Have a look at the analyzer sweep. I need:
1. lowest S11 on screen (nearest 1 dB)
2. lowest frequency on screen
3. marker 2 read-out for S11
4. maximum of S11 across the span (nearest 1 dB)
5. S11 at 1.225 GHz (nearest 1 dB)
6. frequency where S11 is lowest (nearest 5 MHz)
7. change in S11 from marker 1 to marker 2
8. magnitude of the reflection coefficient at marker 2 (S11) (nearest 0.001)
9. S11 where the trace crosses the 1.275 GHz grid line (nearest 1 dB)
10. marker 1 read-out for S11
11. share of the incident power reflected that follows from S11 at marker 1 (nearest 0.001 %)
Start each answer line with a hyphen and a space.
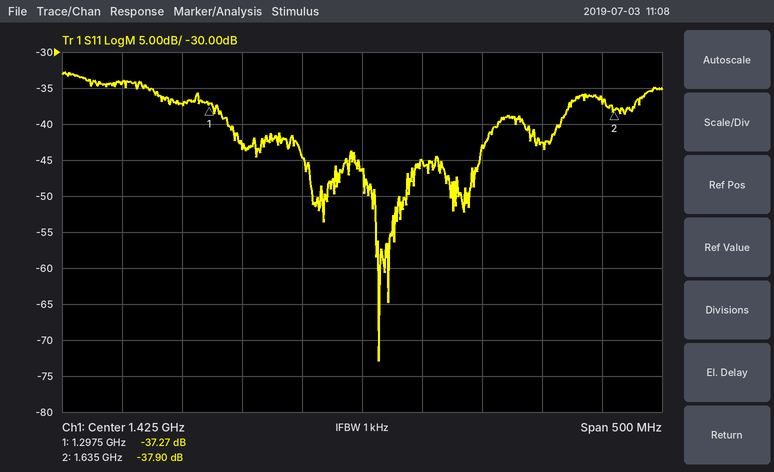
- -73 dB
- 1.175 GHz
- -37.90 dB
- -33 dB
- -34 dB
- 1.440 GHz
- -0.63 dB
- 0.013
- -37 dB
- -37.27 dB
- 0.019 %
